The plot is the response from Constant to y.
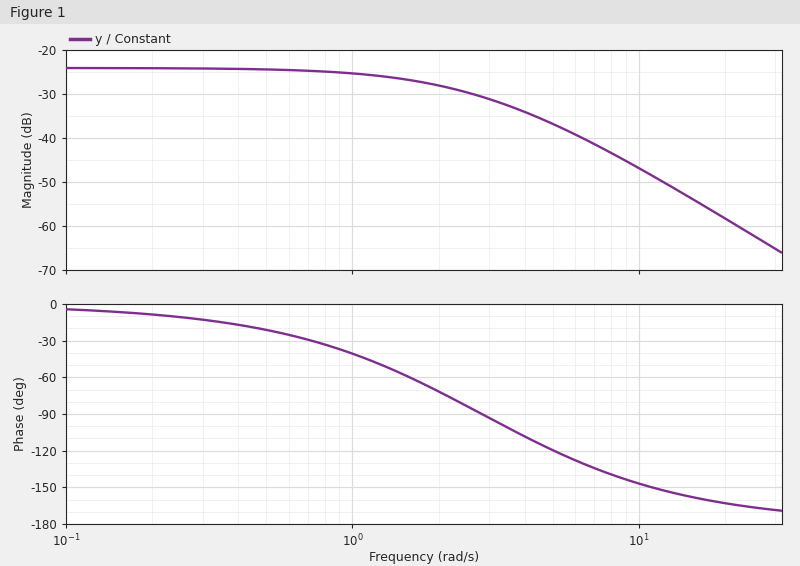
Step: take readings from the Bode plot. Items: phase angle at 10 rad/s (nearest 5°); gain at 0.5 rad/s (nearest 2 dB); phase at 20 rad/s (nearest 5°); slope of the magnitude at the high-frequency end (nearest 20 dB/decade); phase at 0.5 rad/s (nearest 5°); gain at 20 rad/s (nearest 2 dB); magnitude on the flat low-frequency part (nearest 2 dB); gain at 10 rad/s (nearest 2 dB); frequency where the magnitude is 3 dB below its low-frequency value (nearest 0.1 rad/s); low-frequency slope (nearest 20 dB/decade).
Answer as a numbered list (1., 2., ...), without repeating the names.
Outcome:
1. -145°
2. -24 dB
3. -165°
4. -40 dB/decade
5. -20°
6. -58 dB
7. -24 dB
8. -46 dB
9. 1.7 rad/s
10. 0 dB/decade
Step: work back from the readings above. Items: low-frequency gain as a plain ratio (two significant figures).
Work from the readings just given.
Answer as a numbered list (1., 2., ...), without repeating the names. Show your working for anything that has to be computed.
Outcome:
1. 10^(-24 / 20) = 0.063
